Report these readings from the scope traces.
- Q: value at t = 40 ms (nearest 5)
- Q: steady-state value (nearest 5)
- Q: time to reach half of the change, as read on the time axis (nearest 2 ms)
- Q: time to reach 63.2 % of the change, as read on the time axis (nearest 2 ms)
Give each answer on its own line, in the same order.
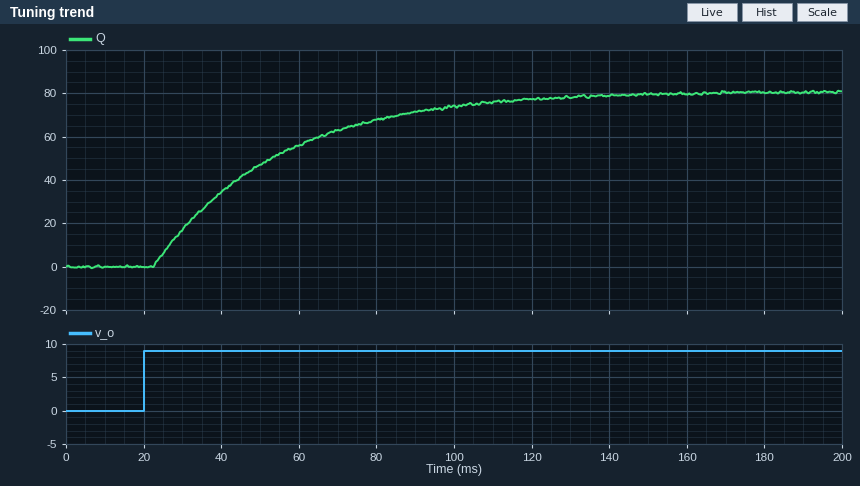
35
80
44 ms
54 ms
